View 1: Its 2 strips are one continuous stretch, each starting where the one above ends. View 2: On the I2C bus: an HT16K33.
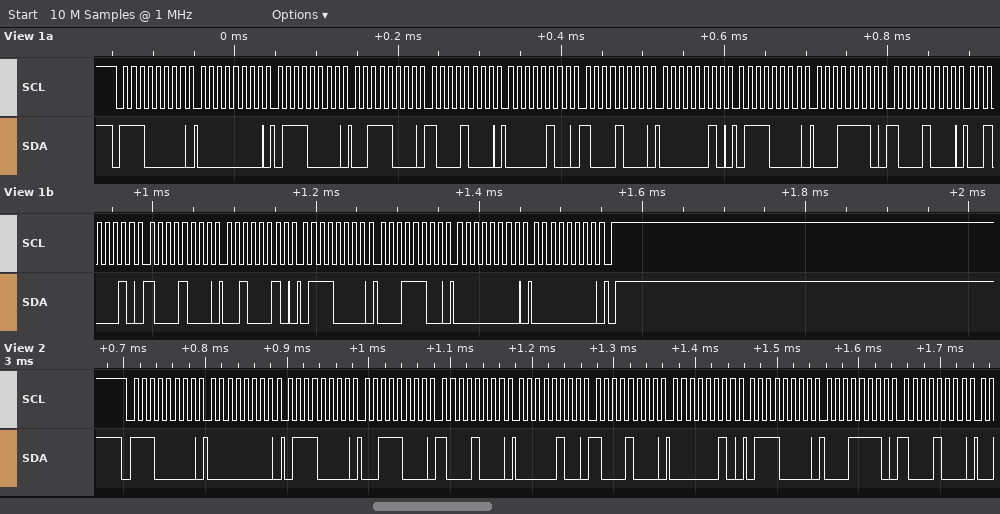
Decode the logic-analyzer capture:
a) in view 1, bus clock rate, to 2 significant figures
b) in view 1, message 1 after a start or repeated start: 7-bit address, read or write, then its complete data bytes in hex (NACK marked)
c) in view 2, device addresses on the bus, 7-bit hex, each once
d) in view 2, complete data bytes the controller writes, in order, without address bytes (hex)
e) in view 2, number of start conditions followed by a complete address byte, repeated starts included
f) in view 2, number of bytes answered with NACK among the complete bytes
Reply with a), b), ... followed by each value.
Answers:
a) 100 kHz
b) 0x70 write: 00 70 38 88 04 88 02 70 1E 88 22 88 22 70 1C 00 00
c) 0x70
d) 00 70 38 88 04 88 02 70 1E 88
e) 1
f) 0
